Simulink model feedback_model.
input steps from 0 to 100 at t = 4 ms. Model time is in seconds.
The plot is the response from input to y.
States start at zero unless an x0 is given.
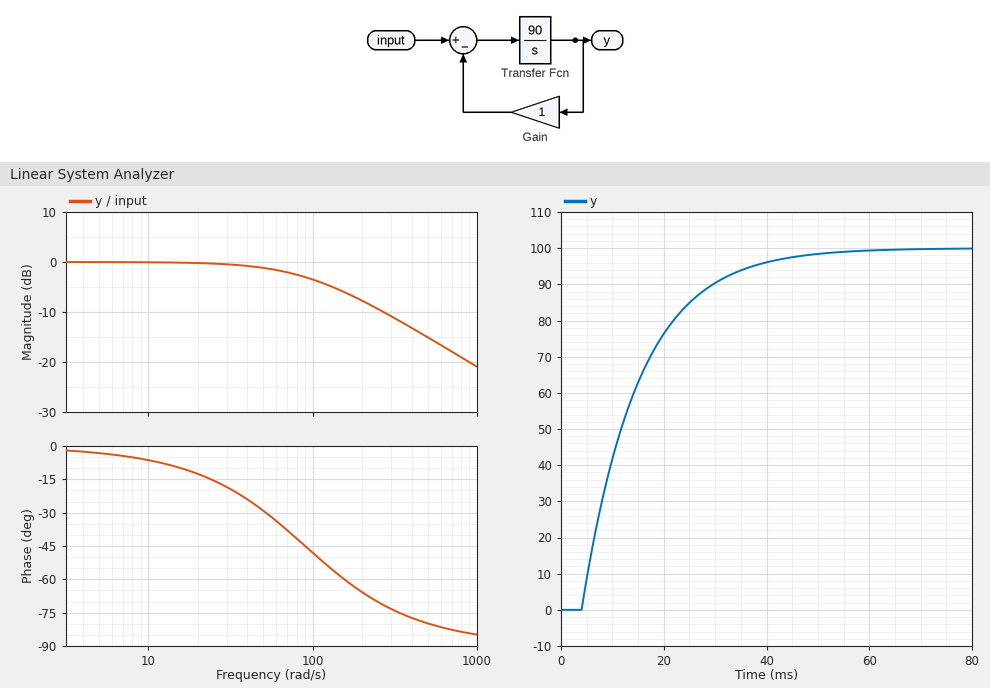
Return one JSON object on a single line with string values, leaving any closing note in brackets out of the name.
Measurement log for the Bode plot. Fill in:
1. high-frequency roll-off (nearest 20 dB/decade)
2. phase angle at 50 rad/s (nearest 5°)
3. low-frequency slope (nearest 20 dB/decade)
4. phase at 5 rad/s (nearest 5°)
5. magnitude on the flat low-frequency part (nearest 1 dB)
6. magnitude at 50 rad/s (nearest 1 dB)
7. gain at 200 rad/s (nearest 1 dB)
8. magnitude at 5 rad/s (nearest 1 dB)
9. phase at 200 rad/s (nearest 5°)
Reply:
{"high-frequency roll-off": "-20 dB/decade", "phase angle at 50 rad/s": "-30°", "low-frequency slope": "0 dB/decade", "phase at 5 rad/s": "-5°", "magnitude on the flat low-frequency part": "0 dB", "magnitude at 50 rad/s": "-1 dB", "gain at 200 rad/s": "-8 dB", "magnitude at 5 rad/s": "0 dB", "phase at 200 rad/s": "-65°"}
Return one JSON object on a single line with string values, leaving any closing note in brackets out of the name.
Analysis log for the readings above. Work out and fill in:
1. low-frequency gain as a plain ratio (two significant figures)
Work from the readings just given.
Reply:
{"low-frequency gain as a plain ratio": "1.0"}
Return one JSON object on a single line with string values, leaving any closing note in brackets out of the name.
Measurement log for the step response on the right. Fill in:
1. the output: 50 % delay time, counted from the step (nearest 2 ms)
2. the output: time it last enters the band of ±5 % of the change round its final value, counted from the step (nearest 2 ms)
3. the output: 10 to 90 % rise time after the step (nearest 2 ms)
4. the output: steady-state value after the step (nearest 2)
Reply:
{"the output: 50 % delay time, counted from the step": "8 ms", "the output: time it last enters the band of ±5 % of the change round its final value, counted from the step": "34 ms", "the output: 10 to 90 % rise time after the step": "24 ms", "the output: steady-state value after the step": "100"}
